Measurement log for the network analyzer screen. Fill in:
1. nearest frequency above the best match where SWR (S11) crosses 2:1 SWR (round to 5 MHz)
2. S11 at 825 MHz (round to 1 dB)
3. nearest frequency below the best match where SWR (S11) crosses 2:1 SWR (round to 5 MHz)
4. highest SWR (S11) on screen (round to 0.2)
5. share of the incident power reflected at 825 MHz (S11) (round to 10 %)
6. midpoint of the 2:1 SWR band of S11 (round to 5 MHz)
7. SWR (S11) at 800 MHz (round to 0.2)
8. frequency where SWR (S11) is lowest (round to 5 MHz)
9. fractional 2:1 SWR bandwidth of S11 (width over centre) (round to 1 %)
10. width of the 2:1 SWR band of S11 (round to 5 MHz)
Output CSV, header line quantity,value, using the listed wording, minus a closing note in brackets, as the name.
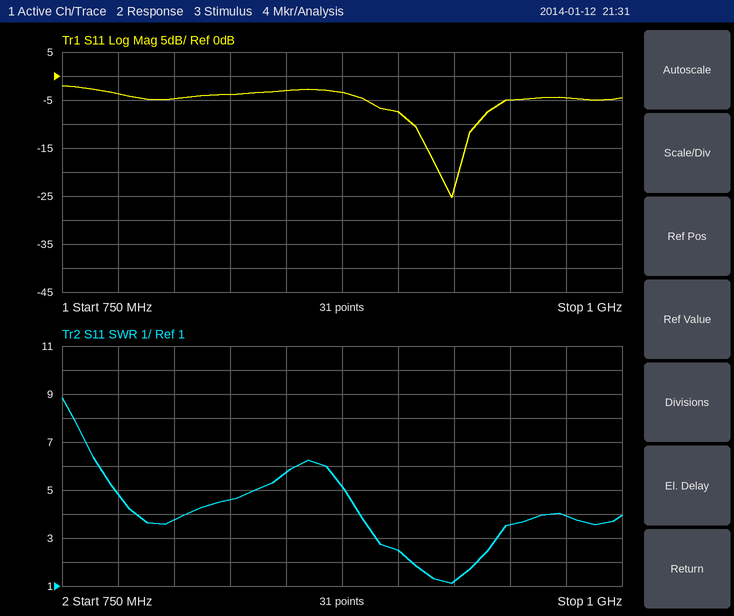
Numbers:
quantity,value
nearest frequency above the best match where SWR (S11) crosses 2:1 SWR,935 MHz
S11 at 825 MHz,-4 dB
nearest frequency below the best match where SWR (S11) crosses 2:1 SWR,905 MHz
highest SWR (S11) on screen,8.8
share of the incident power reflected at 825 MHz (S11),40 %
midpoint of the 2:1 SWR band of S11,920 MHz
SWR (S11) at 800 MHz,3.8
frequency where SWR (S11) is lowest,925 MHz
fractional 2:1 SWR bandwidth of S11 (width over centre),3 %
width of the 2:1 SWR band of S11,30 MHz
